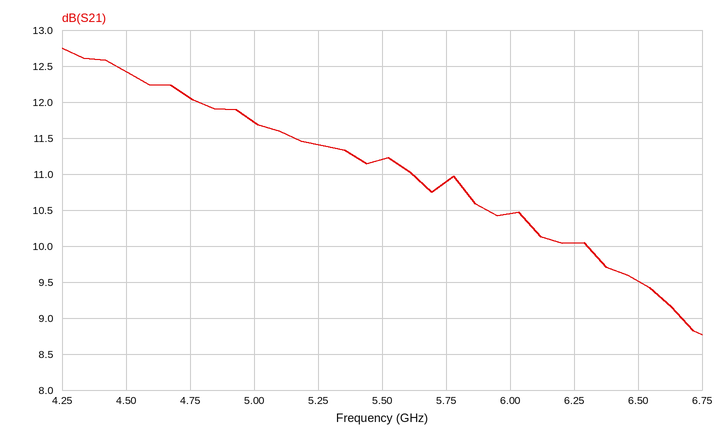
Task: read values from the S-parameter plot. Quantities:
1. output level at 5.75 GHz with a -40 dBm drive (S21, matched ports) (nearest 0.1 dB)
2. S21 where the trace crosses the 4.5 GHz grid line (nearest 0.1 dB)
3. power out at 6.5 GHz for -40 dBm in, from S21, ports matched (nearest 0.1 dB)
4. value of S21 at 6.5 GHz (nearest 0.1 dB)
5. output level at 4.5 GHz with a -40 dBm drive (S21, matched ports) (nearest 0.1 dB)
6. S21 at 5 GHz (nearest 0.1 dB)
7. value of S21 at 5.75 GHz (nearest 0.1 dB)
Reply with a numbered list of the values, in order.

1. -29.1 dBm
2. 12.4 dB
3. -30.5 dBm
4. 9.5 dB
5. -27.6 dBm
6. 11.7 dB
7. 10.9 dB
